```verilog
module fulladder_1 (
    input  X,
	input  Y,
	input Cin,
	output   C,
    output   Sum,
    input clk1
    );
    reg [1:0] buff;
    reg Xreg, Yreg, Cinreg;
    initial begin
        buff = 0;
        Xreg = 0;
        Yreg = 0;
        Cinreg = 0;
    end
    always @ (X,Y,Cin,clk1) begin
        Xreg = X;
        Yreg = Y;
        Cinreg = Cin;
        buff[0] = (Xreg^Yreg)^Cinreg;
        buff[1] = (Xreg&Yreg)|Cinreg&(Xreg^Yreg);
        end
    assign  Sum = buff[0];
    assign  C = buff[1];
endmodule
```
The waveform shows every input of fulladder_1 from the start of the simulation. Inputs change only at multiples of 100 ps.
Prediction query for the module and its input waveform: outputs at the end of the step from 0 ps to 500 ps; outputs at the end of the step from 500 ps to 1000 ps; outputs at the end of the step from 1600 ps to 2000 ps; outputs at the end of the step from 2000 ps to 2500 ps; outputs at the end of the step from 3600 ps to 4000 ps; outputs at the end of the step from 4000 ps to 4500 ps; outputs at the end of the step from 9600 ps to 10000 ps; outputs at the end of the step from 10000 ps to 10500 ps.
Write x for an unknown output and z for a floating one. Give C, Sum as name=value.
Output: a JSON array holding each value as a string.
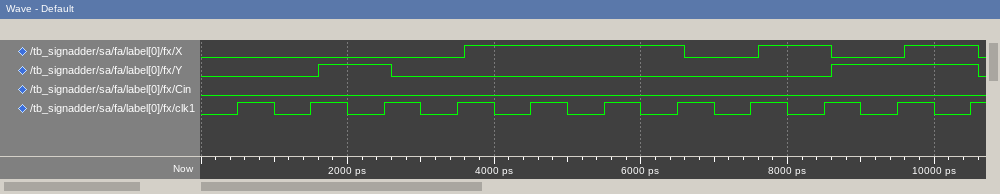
["C=0, Sum=0", "C=0, Sum=0", "C=0, Sum=1", "C=0, Sum=1", "C=0, Sum=1", "C=0, Sum=1", "C=1, Sum=0", "C=1, Sum=0"]
